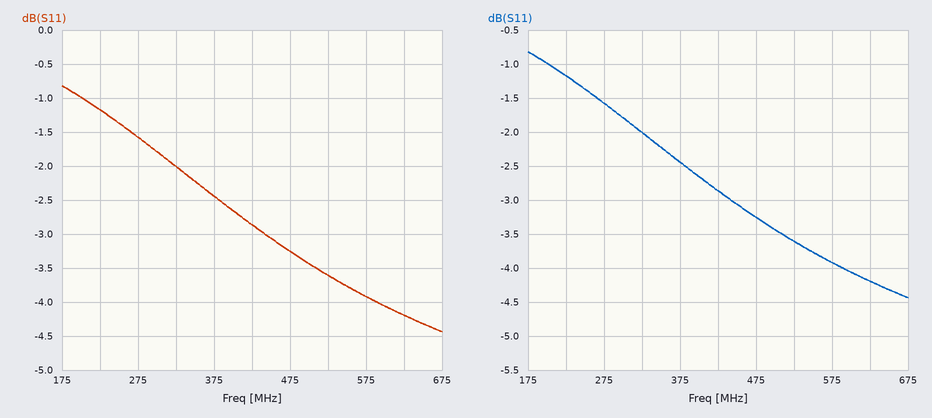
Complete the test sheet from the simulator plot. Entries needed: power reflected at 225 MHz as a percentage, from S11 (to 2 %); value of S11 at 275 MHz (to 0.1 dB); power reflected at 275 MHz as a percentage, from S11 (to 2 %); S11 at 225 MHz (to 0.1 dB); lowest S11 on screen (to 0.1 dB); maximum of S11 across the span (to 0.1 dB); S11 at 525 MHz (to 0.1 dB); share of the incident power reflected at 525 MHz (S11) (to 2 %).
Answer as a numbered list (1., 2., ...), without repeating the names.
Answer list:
1. 76 %
2. -1.6 dB
3. 70 %
4. -1.2 dB
5. -4.4 dB
6. -0.8 dB
7. -3.6 dB
8. 44 %
